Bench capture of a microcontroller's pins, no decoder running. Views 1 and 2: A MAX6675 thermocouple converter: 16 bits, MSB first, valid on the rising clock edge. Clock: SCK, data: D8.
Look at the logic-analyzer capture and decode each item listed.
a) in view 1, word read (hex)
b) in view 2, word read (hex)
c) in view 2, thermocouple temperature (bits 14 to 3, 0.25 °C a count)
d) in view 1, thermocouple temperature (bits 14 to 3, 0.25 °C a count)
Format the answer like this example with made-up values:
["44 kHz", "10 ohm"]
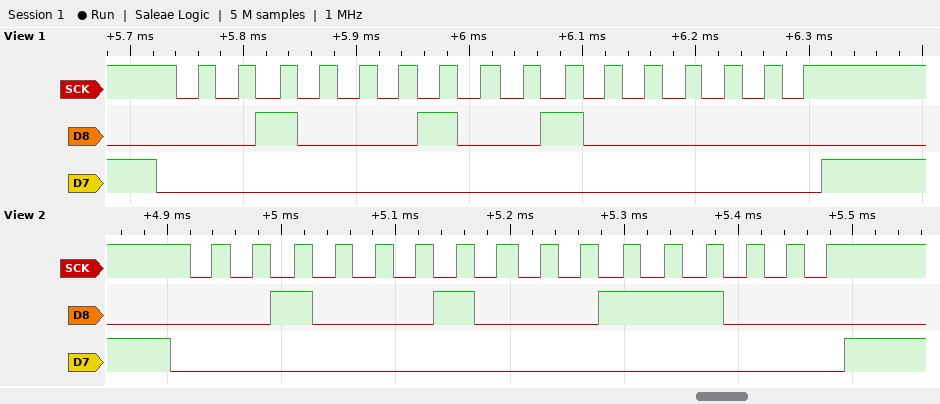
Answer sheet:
["0x2240", "0x2238", "273.75 °C", "274.00 °C"]
